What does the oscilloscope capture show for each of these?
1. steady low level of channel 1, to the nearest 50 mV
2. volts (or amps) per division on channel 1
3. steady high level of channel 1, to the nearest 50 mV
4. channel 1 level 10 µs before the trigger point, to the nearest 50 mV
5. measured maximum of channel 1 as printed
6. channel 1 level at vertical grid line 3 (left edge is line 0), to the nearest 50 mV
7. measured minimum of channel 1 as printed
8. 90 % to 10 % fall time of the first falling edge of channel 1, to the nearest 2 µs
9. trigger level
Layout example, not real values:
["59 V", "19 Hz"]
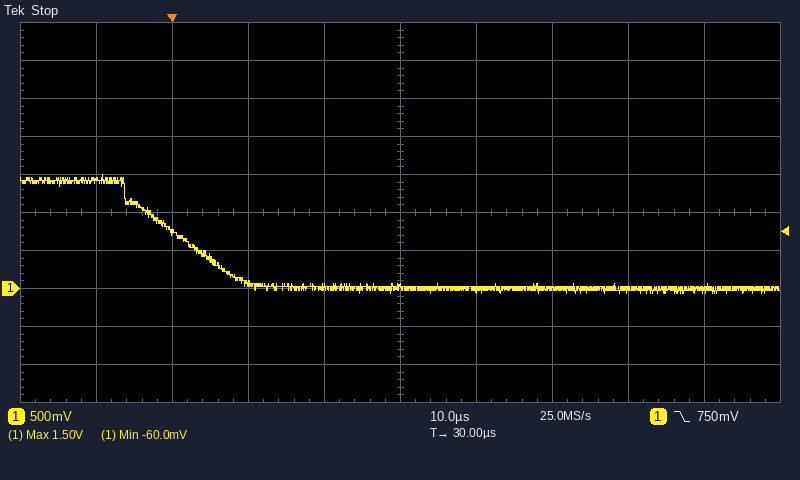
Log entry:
["0 mV", "500 mV", "1.40 V", "1.40 V", "1.50 V", "50 mV", "-60.0 mV", "14 µs", "750 mV"]
